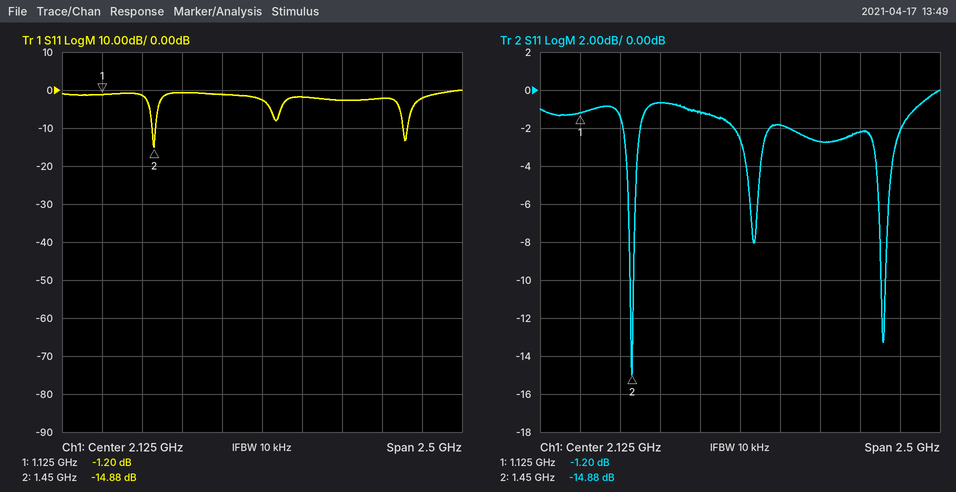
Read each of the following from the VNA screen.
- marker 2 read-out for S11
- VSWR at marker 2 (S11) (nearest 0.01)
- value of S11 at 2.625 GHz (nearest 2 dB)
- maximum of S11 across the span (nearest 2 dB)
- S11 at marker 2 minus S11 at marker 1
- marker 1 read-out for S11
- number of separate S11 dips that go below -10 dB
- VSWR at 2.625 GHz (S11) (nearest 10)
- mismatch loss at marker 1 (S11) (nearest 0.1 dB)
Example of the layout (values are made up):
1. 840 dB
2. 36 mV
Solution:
1. -14.88 dB
2. 1.44
3. -2 dB
4. 0 dB
5. -13.68 dB
6. -1.20 dB
7. 2
8. 10
9. 6.2 dB
